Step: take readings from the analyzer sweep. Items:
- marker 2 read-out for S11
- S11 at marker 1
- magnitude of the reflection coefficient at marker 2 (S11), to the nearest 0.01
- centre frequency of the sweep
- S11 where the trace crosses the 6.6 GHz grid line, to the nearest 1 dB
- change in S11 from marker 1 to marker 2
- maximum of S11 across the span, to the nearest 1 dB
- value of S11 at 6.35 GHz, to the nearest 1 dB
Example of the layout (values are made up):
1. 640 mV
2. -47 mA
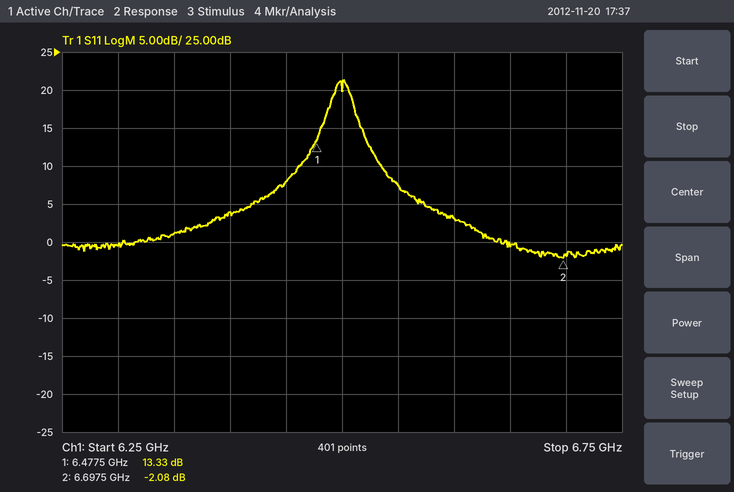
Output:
1. -2.08 dB
2. 13.33 dB
3. 0.79
4. 6.5 GHz
5. 3 dB
6. -15.41 dB
7. 21 dB
8. 1 dB
